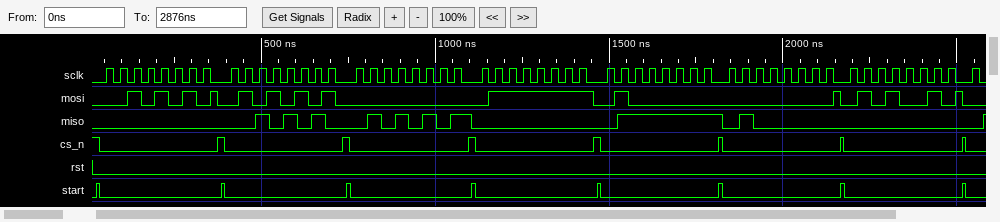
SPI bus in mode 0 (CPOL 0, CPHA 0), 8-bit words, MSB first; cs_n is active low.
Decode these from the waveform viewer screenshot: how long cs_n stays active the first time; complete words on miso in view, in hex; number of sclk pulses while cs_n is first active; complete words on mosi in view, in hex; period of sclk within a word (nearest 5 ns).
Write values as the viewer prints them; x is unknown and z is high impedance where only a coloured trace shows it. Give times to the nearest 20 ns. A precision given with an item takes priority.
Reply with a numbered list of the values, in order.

1. 340 ns
2. 00, 2A, 55, 00, 7F, 40, 00
3. 8
4. 2A, 55, 00, 7F, 40, 00, 52
5. 40 ns
